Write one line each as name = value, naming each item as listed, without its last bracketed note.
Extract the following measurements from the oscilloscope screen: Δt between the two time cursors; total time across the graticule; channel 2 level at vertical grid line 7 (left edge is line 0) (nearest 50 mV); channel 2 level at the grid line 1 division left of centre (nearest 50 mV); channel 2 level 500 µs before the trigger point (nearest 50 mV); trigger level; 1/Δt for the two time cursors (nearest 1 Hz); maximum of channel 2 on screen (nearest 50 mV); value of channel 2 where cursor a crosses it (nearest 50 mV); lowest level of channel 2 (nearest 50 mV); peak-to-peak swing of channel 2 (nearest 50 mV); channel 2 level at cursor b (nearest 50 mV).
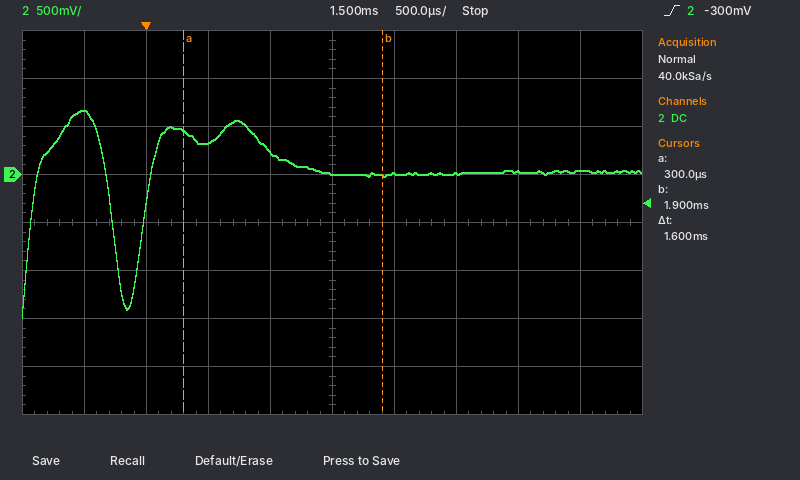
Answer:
Δt between the two time cursors = 1.6 ms
total time across the graticule = 5 ms
channel 2 level at vertical grid line 7 (left edge is line 0) = 0 mV
channel 2 level at the grid line 1 division left of centre = 250 mV
channel 2 level 500 µs before the trigger point = 650 mV
trigger level = -300 mV
1/Δt for the two time cursors = 625 Hz
maximum of channel 2 on screen = 650 mV
value of channel 2 where cursor a crosses it = 450 mV
lowest level of channel 2 = -1.50 V
peak-to-peak swing of channel 2 = 2.15 V
channel 2 level at cursor b = 0 mV
